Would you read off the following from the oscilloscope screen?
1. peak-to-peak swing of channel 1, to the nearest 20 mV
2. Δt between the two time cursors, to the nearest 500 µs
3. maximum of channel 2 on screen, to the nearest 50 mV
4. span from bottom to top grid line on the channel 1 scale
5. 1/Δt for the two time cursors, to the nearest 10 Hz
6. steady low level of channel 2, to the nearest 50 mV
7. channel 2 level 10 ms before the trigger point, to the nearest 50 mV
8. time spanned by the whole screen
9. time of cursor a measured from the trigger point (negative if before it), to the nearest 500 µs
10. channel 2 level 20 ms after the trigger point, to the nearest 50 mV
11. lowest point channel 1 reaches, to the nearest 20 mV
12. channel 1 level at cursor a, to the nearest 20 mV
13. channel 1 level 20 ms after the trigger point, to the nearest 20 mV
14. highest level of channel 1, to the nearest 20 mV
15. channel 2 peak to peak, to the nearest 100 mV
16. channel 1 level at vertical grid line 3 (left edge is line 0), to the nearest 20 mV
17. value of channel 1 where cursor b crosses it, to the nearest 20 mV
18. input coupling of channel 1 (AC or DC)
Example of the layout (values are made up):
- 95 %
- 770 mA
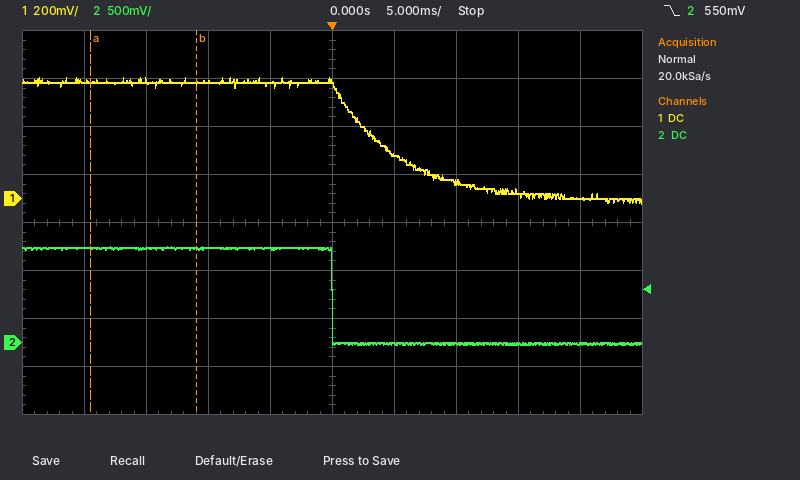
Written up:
- 520 mV
- 8.5 ms
- 1.00 V
- 1.6 V
- 120 Hz
- 0 mV
- 1.00 V
- 50 ms
- -19.5 ms
- 0 mV
- -20 mV
- 480 mV
- 0 mV
- 500 mV
- 1.00 V
- 480 mV
- 480 mV
- DC
